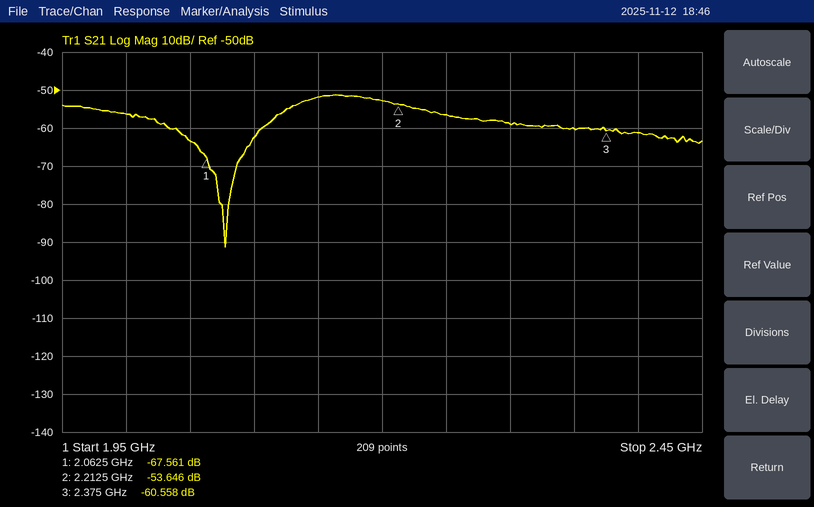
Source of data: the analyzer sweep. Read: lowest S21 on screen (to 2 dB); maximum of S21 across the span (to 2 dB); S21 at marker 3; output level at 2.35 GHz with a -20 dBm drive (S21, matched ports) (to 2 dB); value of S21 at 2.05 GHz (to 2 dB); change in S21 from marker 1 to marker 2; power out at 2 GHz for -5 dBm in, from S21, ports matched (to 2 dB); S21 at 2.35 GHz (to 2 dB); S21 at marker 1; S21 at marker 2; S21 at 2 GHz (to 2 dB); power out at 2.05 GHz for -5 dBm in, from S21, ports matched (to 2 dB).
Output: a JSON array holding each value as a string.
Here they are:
["-92 dB", "-52 dB", "-60.558 dB", "-80 dBm", "-64 dB", "13.915 dB", "-62 dBm", "-60 dB", "-67.561 dB", "-53.646 dB", "-56 dB", "-68 dBm"]
